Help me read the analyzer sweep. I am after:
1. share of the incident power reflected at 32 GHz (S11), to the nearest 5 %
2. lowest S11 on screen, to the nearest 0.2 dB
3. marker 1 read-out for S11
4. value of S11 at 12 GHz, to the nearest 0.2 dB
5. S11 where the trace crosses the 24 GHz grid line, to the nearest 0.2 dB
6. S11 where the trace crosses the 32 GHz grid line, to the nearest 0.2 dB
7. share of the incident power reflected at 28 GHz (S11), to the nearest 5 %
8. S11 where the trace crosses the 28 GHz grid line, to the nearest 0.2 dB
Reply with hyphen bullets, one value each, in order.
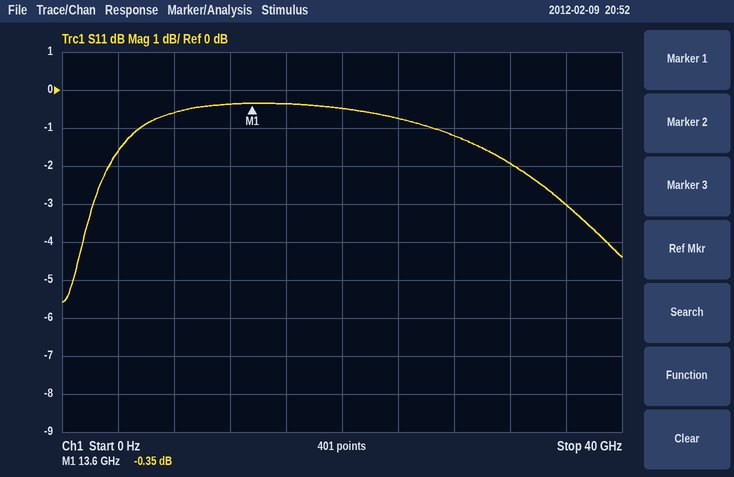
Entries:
- 65 %
- -5.6 dB
- -0.35 dB
- -0.4 dB
- -0.8 dB
- -2.0 dB
- 75 %
- -1.2 dB
